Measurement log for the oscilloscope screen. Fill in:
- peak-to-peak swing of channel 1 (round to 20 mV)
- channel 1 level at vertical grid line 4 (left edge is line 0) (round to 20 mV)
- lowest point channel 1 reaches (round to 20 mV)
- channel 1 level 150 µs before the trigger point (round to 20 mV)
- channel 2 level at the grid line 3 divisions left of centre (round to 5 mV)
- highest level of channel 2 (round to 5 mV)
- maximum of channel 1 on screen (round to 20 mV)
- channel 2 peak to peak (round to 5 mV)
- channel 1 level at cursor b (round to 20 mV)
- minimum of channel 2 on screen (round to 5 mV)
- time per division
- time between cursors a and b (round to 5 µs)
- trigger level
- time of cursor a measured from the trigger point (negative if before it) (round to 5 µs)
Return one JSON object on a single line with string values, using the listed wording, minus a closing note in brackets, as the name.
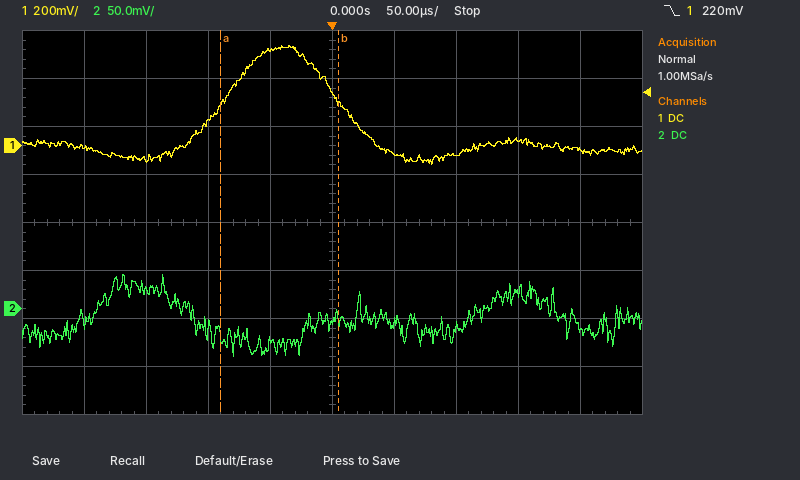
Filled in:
{"peak-to-peak swing of channel 1": "500 mV", "channel 1 level at vertical grid line 4 (left edge is line 0)": "400 mV", "lowest point channel 1 reaches": "-80 mV", "channel 1 level 150 µs before the trigger point": "-60 mV", "channel 2 level at the grid line 3 divisions left of centre": "20 mV", "highest level of channel 2": "35 mV", "maximum of channel 1 on screen": "420 mV", "channel 2 peak to peak": "85 mV", "channel 1 level at cursor b": "180 mV", "minimum of channel 2 on screen": "-50 mV", "time per division": "50 µs", "time between cursors a and b": "95 µs", "trigger level": "220 mV", "time of cursor a measured from the trigger point (negative if before it)": "-90 µs"}
